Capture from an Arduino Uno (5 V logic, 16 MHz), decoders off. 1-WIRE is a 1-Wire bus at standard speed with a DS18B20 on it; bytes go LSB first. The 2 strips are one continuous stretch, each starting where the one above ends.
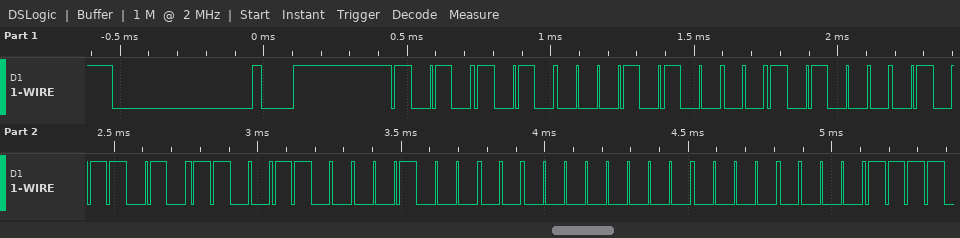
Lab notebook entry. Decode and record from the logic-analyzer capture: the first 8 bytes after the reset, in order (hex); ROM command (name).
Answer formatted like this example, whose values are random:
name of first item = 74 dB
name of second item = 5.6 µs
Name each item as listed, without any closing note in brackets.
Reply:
the first 8 bytes after the reset, in order = 55 28 14 5A 33 04 00 00
ROM command = Match ROM
